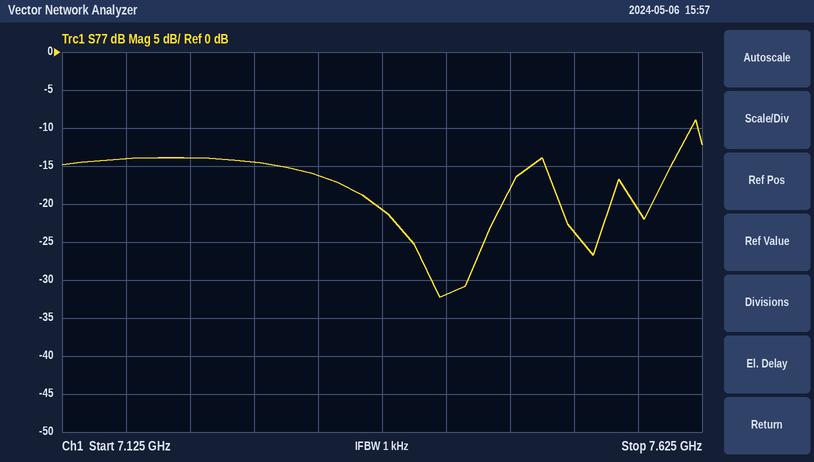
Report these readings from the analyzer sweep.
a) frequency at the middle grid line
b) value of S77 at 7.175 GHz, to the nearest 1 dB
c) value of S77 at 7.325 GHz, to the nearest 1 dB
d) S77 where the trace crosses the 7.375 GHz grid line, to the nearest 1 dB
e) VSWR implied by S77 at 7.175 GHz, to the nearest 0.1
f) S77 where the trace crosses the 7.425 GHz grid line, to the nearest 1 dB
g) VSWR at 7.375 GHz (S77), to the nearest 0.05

7.375 GHz
-14 dB
-16 dB
-21 dB
1.5
-32 dB
1.20
